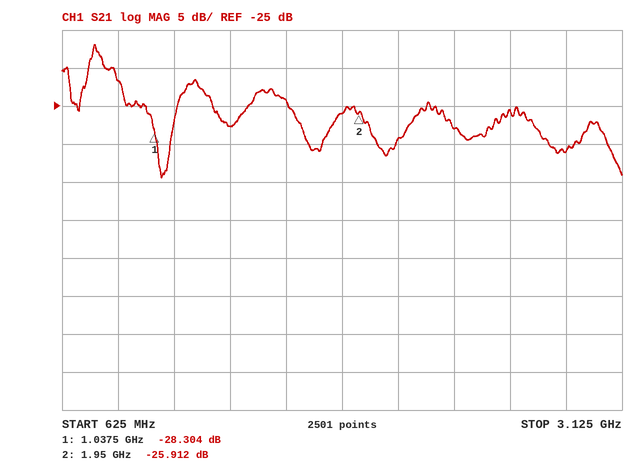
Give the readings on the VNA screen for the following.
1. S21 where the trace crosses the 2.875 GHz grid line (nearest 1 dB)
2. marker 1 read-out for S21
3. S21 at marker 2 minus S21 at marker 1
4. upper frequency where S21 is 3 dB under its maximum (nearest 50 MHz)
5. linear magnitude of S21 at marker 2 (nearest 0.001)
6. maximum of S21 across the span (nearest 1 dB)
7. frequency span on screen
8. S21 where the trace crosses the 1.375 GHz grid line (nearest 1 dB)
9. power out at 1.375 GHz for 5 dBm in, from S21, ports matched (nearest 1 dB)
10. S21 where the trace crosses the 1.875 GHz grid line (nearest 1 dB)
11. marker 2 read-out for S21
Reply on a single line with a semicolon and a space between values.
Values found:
-31 dB; -28.304 dB; 2.392 dB; 800 MHz; 0.051; -17 dB; 2.5 GHz; -28 dB; -23 dBm; -26 dB; -25.912 dB
